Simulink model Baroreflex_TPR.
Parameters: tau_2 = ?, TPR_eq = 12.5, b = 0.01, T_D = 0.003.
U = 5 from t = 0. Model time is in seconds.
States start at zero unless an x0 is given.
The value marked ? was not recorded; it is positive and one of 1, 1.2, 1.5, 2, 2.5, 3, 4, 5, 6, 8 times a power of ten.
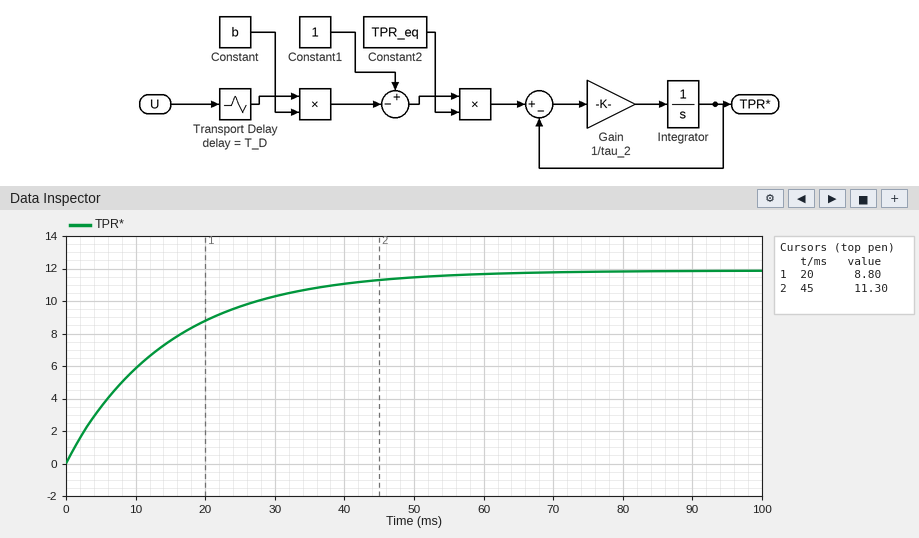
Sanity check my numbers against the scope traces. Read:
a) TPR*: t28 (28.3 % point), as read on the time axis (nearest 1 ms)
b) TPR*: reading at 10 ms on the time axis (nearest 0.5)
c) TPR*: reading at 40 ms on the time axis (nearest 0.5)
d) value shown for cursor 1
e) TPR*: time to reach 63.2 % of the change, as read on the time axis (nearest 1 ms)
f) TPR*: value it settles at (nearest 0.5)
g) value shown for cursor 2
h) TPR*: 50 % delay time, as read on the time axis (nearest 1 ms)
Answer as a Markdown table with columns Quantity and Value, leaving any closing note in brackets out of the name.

| Quantity | Value |
|---|---|
| TPR*: t28 (28.3 % point), as read on the time axis | 5 ms |
| TPR*: reading at 10 ms on the time axis | 6.0 |
| TPR*: reading at 40 ms on the time axis | 11.0 |
| value shown for cursor 1 | 8.80 |
| TPR*: time to reach 63.2 % of the change, as read on the time axis | 15 ms |
| TPR*: value it settles at | 12.0 |
| value shown for cursor 2 | 11.30 |
| TPR*: 50 % delay time, as read on the time axis | 10 ms |
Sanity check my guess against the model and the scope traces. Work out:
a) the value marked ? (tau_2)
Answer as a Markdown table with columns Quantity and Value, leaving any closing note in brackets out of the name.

| Quantity | Value |
|---|---|
| the value marked ? | 0.015 |
